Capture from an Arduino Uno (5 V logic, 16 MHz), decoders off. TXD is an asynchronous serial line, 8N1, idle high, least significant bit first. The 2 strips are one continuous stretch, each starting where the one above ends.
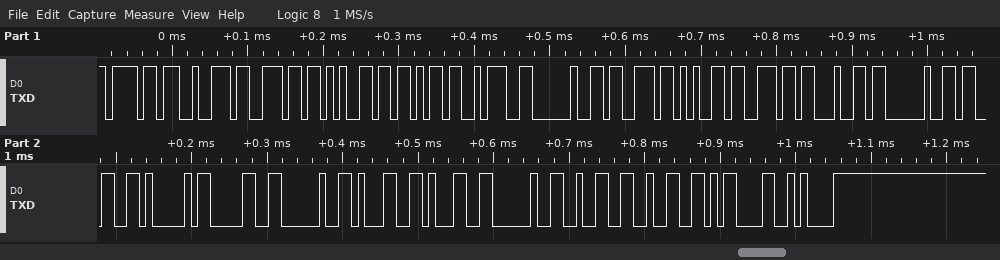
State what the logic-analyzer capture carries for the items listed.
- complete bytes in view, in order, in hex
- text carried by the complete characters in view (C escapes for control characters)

6F 72 6E 65 6B 3A 20 73 65 6E 64 20 33 41 30 20 31 31 20 32 32 0D 0A
"ornek: send 3A0 11 22\r\n"
